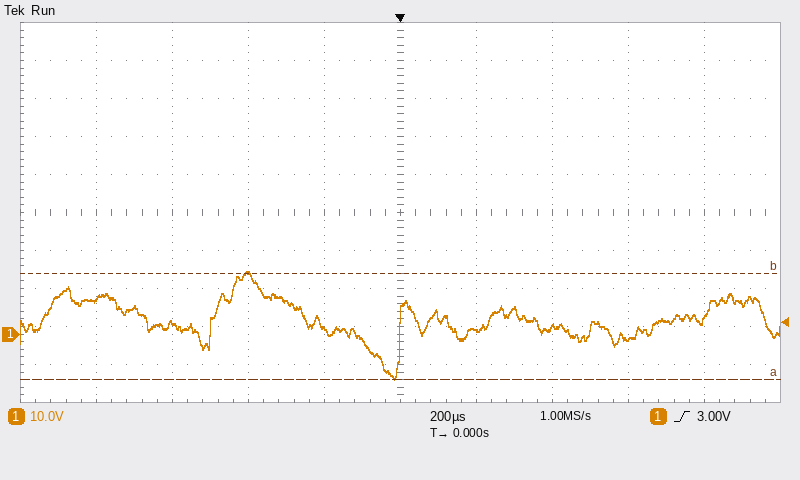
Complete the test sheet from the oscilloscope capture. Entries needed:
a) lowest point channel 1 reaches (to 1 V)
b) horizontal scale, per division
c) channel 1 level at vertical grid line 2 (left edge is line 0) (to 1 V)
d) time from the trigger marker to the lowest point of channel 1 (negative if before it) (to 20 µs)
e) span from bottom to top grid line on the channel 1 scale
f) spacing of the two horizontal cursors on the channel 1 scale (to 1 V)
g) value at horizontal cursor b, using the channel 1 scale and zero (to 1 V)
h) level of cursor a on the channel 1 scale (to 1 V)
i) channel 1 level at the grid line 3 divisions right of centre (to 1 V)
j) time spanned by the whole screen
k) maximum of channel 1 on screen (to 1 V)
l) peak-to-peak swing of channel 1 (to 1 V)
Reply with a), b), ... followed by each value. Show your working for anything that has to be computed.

a) -12 V
b) 200 µs
c) 3 V
d) -20 µs
e) 100 V
f) 28 V
g) 16 V
h) -12 V
i) -1 V
j) 2 ms
k) 16 V
l) 16 V − (-12 V) = 28 V
